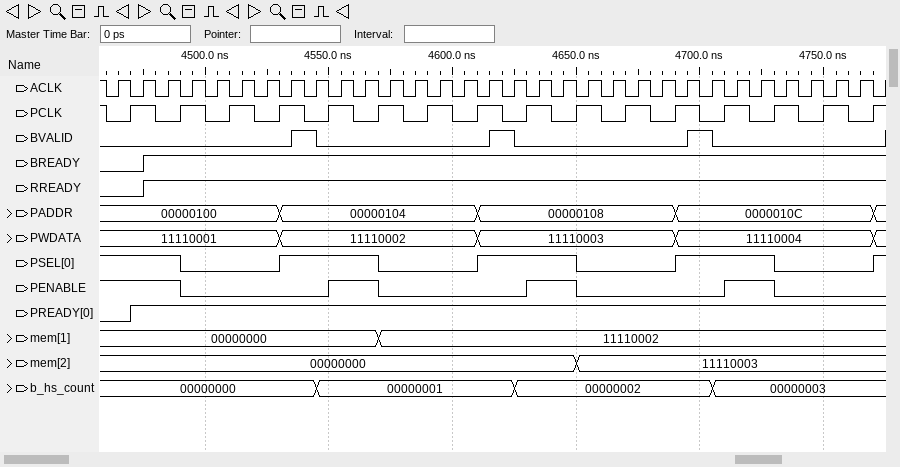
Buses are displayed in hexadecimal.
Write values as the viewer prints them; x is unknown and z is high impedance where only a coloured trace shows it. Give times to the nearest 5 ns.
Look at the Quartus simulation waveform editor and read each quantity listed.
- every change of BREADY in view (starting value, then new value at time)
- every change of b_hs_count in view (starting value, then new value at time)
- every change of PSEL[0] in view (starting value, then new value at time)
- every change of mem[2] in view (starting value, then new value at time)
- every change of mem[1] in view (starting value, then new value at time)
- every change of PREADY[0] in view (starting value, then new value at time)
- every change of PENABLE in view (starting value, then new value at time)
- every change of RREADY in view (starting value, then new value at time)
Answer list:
0, 1 at 4475 ns
00000000, 00000001 at 4545 ns, 00000002 at 4625 ns, 00000003 at 4705 ns
1, 0 at 4490 ns, 1 at 4530 ns, 0 at 4570 ns, 1 at 4610 ns, 0 at 4650 ns, 1 at 4690 ns, 0 at 4730 ns, 1 at 4770 ns
00000000, 11110003 at 4650 ns
00000000, 11110002 at 4570 ns
0, 1 at 4470 ns
1, 0 at 4490 ns, 1 at 4550 ns, 0 at 4570 ns, 1 at 4630 ns, 0 at 4650 ns, 1 at 4710 ns, 0 at 4730 ns
0, 1 at 4475 ns
